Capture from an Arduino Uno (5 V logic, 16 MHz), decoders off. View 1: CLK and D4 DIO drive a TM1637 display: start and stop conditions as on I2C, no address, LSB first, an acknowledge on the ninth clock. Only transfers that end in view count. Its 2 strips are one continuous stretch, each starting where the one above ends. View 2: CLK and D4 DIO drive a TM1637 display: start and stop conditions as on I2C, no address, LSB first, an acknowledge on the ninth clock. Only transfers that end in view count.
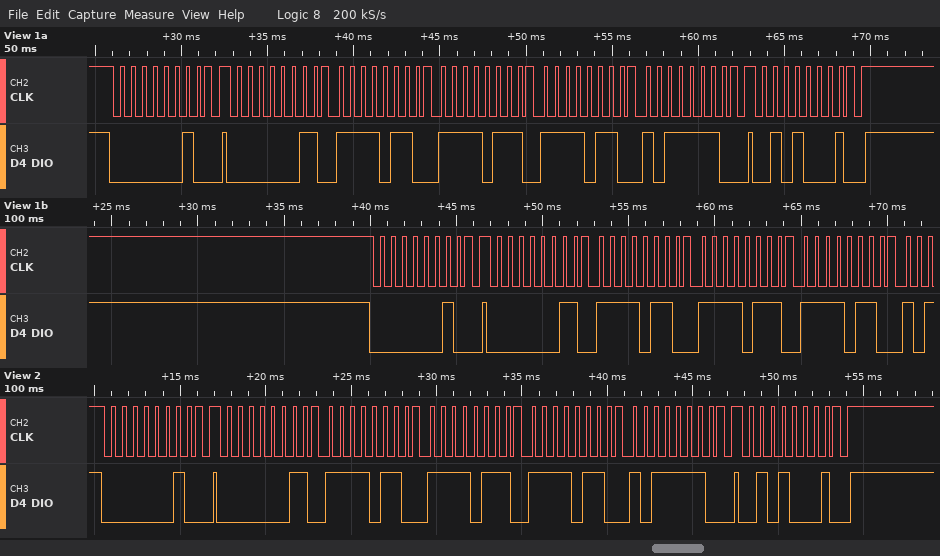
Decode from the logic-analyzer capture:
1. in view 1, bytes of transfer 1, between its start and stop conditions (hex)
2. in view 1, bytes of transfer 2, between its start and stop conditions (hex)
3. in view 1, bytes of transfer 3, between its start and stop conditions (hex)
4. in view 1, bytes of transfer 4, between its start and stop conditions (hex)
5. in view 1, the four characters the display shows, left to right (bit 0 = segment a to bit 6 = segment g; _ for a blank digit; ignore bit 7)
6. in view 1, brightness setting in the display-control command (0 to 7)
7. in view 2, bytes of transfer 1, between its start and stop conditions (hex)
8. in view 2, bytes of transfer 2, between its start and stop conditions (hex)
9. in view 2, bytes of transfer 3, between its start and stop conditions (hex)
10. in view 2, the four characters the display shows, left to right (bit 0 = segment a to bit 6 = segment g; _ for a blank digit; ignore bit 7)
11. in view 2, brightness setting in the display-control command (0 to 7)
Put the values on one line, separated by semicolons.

40; C0 6F EF 6F 7D; 8A; 40; 9996; 2; 40; C0 6F EF 6F 7D; 8A; 9996; 2
